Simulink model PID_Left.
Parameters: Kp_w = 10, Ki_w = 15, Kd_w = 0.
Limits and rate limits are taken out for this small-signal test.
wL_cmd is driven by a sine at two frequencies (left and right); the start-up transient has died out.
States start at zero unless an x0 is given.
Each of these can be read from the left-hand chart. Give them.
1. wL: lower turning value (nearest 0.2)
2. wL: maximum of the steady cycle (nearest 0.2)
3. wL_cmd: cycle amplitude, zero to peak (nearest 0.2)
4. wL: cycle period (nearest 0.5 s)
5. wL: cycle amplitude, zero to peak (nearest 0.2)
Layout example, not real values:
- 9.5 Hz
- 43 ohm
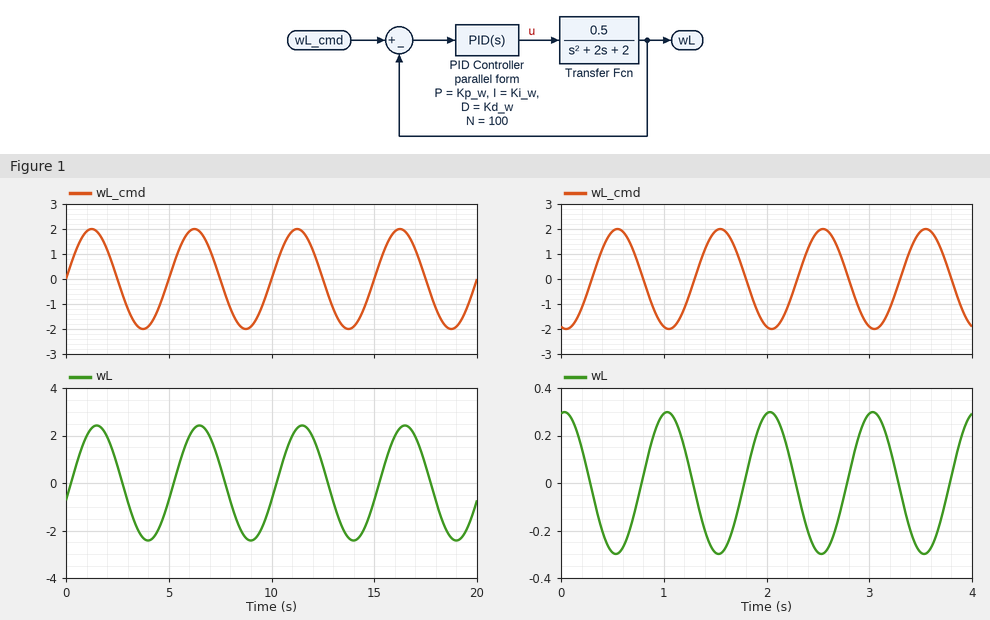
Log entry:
- -2.4
- 2.4
- 2.0
- 5.0 s
- 2.4
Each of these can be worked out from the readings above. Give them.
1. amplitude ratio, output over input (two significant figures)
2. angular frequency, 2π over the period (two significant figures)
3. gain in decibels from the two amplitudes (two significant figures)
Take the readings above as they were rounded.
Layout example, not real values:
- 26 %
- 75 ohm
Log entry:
- 1.2
- 1.3 rad/s
- 1.6 dB
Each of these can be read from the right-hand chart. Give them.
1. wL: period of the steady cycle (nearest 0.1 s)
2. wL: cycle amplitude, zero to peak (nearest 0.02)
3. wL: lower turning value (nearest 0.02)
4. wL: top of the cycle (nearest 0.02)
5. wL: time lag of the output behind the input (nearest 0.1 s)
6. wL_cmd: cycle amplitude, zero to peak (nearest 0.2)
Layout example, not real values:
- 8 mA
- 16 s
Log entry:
- 1.0 s
- 0.30
- -0.30
- 0.30
- 0.5 s
- 2.0
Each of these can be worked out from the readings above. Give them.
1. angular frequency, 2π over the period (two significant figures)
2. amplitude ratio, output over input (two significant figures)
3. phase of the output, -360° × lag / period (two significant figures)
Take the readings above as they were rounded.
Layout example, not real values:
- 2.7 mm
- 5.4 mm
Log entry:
- 6.3 rad/s
- 0.15
- -180°
